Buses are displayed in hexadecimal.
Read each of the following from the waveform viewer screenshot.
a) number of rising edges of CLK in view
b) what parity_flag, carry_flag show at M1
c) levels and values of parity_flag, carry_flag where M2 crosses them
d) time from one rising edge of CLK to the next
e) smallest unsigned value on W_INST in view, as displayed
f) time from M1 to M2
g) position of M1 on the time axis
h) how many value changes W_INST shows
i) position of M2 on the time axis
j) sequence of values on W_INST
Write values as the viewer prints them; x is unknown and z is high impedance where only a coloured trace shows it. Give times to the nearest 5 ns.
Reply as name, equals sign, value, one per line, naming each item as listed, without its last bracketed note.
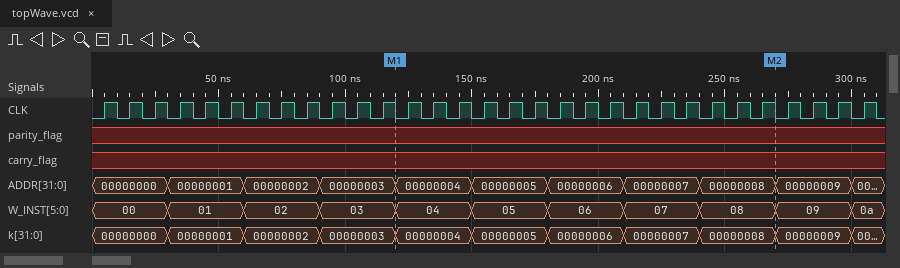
number of rising edges of CLK in view = 31
what parity_flag, carry_flag show at M1 = parity_flag=x, carry_flag=x
levels and values of parity_flag, carry_flag where M2 crosses them = parity_flag=x, carry_flag=x
time from one rising edge of CLK to the next = 10 ns
smallest unsigned value on W_INST in view, as displayed = 00
time from M1 to M2 = 150 ns
position of M1 on the time axis = 120 ns
how many value changes W_INST shows = 10
position of M2 on the time axis = 270 ns
sequence of values on W_INST = 00, 01, 02, 03, 04, 05, 06, 07, 08, 09, 0a
